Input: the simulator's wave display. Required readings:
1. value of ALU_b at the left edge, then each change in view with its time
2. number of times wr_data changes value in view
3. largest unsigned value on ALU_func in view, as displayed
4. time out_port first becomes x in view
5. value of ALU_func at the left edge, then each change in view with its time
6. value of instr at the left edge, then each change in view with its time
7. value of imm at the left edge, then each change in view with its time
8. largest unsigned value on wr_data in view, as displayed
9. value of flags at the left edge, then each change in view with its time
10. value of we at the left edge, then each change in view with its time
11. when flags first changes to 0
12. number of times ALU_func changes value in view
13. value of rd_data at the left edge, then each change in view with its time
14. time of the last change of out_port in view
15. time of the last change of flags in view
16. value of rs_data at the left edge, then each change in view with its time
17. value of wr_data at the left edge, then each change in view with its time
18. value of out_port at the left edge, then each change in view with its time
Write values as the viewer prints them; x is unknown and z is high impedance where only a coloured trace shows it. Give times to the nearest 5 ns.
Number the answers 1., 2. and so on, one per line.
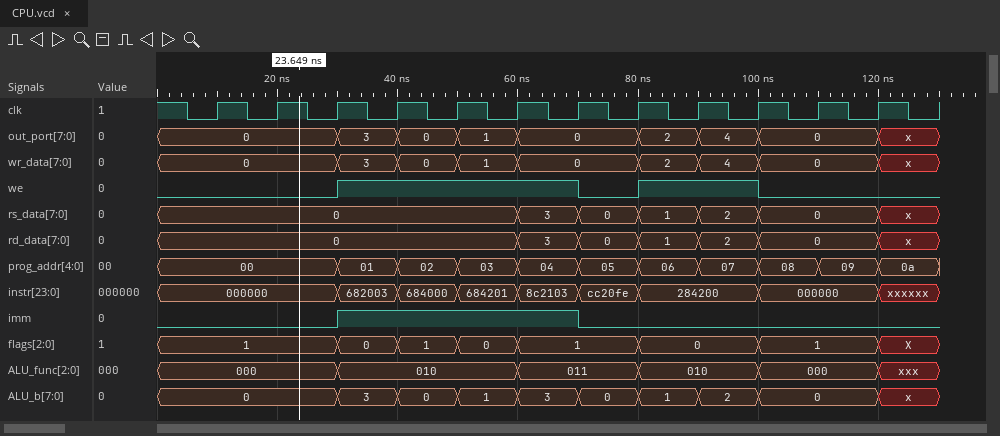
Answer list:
1. 0, 3 at 30 ns, 0 at 40 ns, 1 at 50 ns, 3 at 60 ns, 0 at 70 ns, 1 at 80 ns, 2 at 90 ns, 0 at 100 ns, x at 120 ns
2. 8
3. 011
4. 120 ns
5. 000, 010 at 30 ns, 011 at 60 ns, 010 at 80 ns, 000 at 100 ns, xxx at 120 ns
6. 000000, 682003 at 30 ns, 684000 at 40 ns, 684201 at 50 ns, 8c2103 at 60 ns, cc20fe at 70 ns, 284200 at 80 ns, 000000 at 100 ns, xxxxxx at 120 ns
7. 0, 1 at 30 ns, 0 at 70 ns
8. 4
9. 1, 0 at 30 ns, 1 at 40 ns, 0 at 50 ns, 1 at 60 ns, 0 at 80 ns, 1 at 100 ns, X at 120 ns
10. 0, 1 at 30 ns, 0 at 70 ns, 1 at 80 ns, 0 at 100 ns
11. 30 ns
12. 5
13. 0, 3 at 60 ns, 0 at 70 ns, 1 at 80 ns, 2 at 90 ns, 0 at 100 ns, x at 120 ns
14. 120 ns
15. 120 ns
16. 0, 3 at 60 ns, 0 at 70 ns, 1 at 80 ns, 2 at 90 ns, 0 at 100 ns, x at 120 ns
17. 0, 3 at 30 ns, 0 at 40 ns, 1 at 50 ns, 0 at 60 ns, 2 at 80 ns, 4 at 90 ns, 0 at 100 ns, x at 120 ns
18. 0, 3 at 30 ns, 0 at 40 ns, 1 at 50 ns, 0 at 60 ns, 2 at 80 ns, 4 at 90 ns, 0 at 100 ns, x at 120 ns
